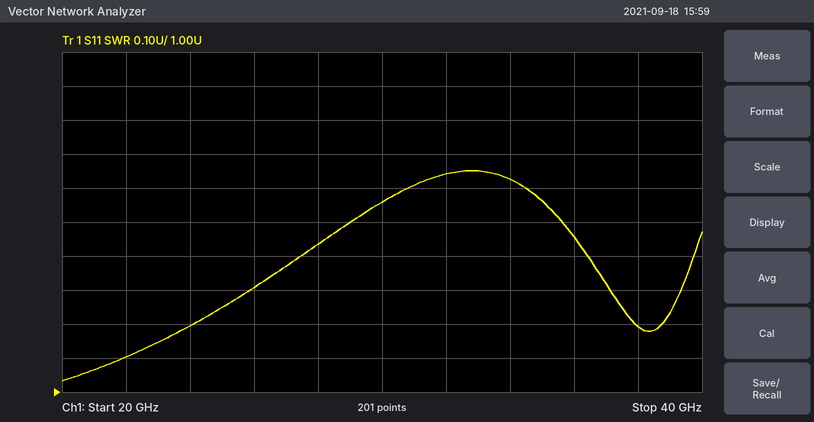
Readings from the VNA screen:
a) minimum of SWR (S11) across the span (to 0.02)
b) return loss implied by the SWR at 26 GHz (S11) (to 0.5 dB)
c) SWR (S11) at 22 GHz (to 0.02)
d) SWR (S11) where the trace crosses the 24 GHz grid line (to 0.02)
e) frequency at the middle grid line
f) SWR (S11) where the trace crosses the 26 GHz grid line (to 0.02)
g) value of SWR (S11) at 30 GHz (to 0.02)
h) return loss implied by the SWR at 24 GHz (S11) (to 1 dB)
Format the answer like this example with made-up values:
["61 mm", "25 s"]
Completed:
["1.04", "17.5 dB", "1.10", "1.20", "30 GHz", "1.30", "1.56", "21 dB"]
